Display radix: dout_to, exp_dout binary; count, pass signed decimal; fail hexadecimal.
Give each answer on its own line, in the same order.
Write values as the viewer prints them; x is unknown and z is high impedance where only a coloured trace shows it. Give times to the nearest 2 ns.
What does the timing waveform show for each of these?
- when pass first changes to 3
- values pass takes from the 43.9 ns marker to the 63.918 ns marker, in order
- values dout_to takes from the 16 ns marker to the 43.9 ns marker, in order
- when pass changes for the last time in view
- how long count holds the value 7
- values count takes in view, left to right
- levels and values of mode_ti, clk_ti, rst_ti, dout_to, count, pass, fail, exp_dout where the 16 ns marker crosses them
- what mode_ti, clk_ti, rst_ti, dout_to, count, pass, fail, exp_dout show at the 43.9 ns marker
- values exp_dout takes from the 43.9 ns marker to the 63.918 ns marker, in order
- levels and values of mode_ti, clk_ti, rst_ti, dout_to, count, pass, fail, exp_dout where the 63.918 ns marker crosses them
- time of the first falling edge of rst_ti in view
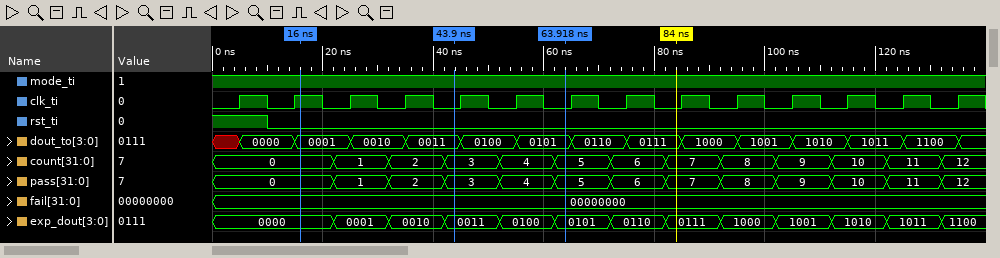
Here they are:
42 ns
3, 4, 5
0001, 0010, 0011
132 ns
10 ns
0, 1, 2, 3, 4, 5, 6, 7, 8, 9, 10, 11, 12
mode_ti=1, clk_ti=1, rst_ti=0, dout_to=0001, count=0, pass=0, fail=00000000, exp_dout=0000
mode_ti=1, clk_ti=0, rst_ti=0, dout_to=0011, count=3, pass=3, fail=00000000, exp_dout=0011
0011, 0100, 0101
mode_ti=1, clk_ti=0, rst_ti=0, dout_to=0101, count=5, pass=5, fail=00000000, exp_dout=0101
10 ns
